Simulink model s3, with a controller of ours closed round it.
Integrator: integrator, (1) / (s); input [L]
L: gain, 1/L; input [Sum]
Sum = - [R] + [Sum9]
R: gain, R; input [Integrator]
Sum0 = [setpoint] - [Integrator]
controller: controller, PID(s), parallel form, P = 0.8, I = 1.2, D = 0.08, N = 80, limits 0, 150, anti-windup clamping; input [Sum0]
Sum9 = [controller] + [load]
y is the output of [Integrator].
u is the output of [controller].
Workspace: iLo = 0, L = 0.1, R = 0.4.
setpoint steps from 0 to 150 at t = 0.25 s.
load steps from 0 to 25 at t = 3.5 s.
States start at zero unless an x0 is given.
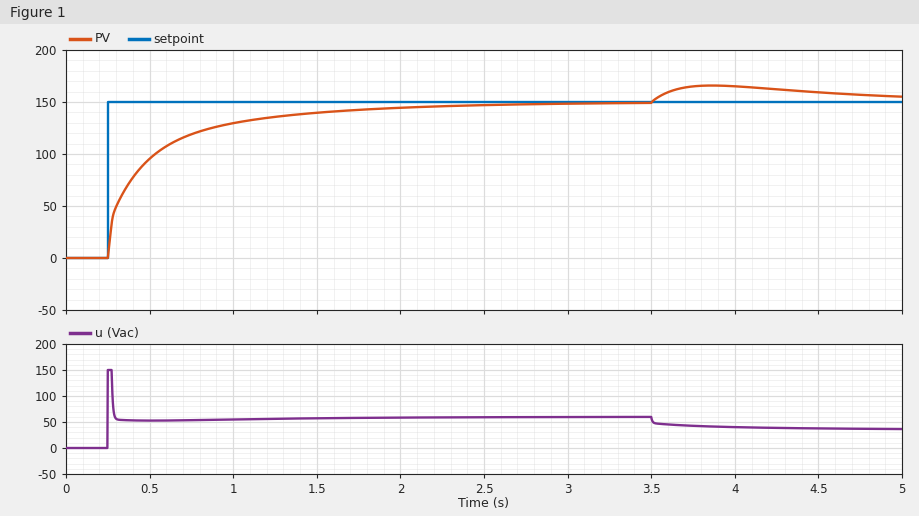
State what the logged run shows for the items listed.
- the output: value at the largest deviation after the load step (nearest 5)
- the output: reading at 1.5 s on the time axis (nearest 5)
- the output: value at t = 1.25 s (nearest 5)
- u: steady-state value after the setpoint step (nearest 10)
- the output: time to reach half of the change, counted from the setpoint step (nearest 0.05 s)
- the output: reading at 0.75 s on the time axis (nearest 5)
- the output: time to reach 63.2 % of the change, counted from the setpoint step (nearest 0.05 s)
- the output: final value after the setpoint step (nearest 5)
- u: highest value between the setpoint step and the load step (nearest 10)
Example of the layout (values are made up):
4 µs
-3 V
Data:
165
140
135
60
0.15 s
120
0.25 s
150
150
